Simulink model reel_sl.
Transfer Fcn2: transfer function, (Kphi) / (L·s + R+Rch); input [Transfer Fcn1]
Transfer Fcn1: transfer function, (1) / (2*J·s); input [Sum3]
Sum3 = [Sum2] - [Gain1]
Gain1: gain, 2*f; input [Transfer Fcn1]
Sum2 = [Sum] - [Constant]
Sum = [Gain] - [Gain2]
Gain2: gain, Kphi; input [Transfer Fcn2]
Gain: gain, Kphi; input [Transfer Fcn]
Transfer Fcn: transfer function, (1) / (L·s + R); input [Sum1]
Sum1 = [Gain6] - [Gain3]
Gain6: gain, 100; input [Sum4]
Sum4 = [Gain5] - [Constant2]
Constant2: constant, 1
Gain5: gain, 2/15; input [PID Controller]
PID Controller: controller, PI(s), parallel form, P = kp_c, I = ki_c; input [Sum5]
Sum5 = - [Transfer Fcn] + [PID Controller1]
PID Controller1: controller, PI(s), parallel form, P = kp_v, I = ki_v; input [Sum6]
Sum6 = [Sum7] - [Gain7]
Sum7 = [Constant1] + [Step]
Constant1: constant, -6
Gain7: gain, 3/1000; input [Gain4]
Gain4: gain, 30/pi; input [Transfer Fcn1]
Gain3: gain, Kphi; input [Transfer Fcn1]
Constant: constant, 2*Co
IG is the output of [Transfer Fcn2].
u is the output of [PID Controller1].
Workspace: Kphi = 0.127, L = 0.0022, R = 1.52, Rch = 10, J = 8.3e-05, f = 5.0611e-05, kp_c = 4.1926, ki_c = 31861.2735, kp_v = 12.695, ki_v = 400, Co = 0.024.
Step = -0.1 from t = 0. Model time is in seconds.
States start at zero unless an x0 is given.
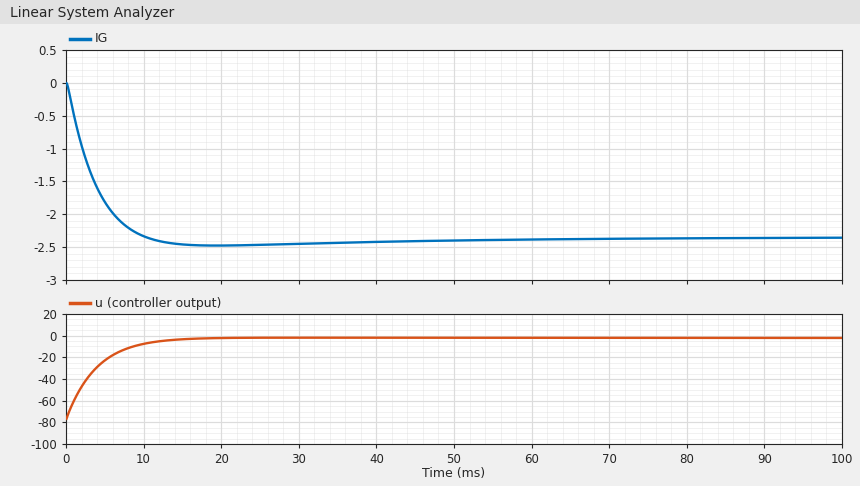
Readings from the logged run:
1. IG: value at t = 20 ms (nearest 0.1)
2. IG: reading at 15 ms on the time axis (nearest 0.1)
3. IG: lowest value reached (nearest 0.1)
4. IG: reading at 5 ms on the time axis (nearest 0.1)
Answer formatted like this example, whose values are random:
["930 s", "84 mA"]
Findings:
["-2.5", "-2.5", "-2.5", "-1.8"]
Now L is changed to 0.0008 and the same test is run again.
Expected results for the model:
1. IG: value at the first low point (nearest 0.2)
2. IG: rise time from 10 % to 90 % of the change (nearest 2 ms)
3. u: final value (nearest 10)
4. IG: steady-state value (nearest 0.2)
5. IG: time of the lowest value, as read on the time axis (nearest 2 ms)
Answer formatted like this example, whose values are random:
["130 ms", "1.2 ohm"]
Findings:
["-2.4", "6 ms", "0", "-2.4", "20 ms"]
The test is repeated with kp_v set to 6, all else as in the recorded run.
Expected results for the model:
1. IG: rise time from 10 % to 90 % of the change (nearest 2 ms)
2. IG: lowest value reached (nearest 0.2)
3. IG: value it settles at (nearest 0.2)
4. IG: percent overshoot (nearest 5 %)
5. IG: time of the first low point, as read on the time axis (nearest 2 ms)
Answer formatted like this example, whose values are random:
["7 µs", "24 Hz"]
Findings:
["10 ms", "-2.8", "-2.4", "15 %", "24 ms"]
